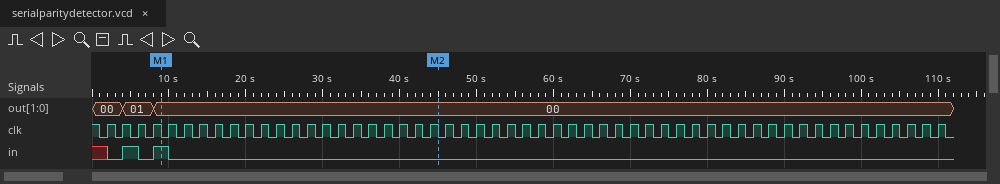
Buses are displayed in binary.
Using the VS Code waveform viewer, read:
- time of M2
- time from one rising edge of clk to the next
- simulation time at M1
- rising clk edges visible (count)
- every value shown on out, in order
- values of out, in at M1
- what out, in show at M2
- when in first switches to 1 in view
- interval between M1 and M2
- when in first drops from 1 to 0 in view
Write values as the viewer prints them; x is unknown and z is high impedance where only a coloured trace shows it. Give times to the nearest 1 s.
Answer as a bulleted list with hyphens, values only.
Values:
- 45 s
- 2 s
- 9 s
- 55
- 00, 01, 00
- out=00, in=1
- out=00, in=0
- 4 s
- 36 s
- 6 s
